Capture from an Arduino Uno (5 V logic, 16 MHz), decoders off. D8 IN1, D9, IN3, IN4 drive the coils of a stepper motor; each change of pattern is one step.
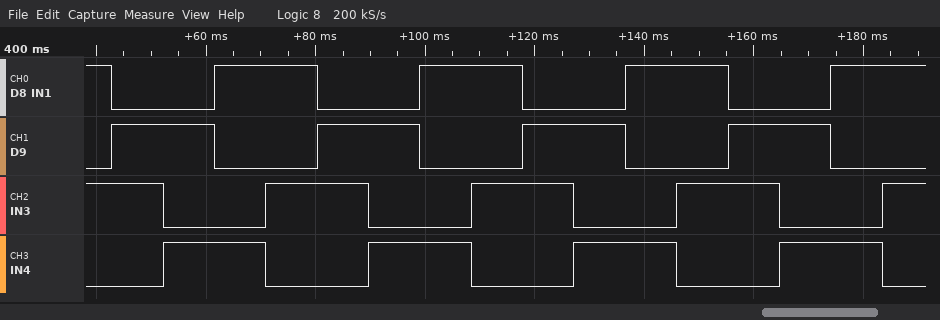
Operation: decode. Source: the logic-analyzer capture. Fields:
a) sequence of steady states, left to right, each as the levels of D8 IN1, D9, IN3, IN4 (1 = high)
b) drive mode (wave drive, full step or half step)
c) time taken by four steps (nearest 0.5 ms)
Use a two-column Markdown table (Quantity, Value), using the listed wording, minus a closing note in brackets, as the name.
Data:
| Quantity | Value |
|---|---|
| sequence of steady states, left to right, each as the levels of D8 IN1, D9, IN3, IN4 | 1010 0110 0101 1001 1010 0110 0101 1001 1010 0110 0101 1001 1010 0110 0101 1001 1010 |
| drive mode | full step |
| time taken by four steps | 37.5 ms |
